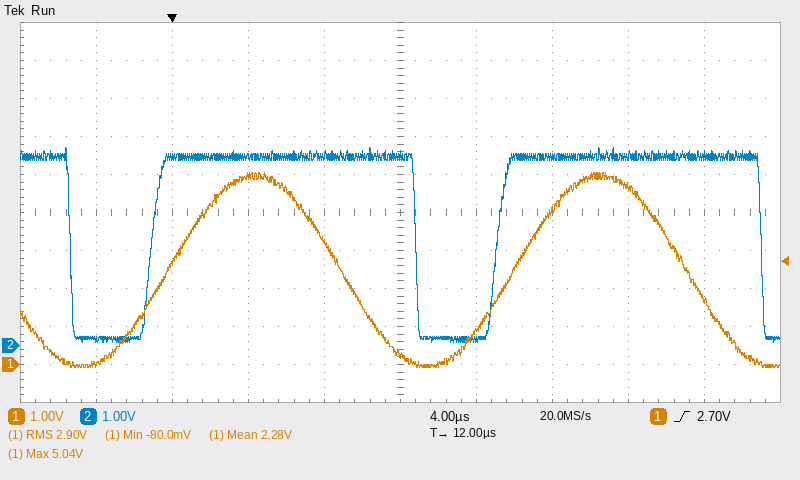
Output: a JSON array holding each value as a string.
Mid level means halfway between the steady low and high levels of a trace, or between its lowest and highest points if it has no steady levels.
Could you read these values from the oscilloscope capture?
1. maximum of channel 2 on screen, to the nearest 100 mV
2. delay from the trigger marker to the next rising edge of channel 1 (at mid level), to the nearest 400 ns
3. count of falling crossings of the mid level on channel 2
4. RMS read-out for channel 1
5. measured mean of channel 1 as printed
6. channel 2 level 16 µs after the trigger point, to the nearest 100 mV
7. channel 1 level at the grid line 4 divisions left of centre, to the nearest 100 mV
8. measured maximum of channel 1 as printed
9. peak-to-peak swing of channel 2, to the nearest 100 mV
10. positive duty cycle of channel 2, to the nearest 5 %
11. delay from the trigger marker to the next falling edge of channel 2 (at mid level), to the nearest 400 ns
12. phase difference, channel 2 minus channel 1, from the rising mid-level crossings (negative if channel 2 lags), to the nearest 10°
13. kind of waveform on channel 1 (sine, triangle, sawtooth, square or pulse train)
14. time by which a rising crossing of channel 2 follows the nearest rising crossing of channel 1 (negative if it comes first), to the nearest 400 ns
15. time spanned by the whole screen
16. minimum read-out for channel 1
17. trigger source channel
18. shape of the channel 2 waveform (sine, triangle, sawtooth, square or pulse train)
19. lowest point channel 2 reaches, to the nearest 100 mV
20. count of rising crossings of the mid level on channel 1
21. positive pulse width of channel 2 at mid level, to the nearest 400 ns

["5.2 V", "18.0 µs", "3", "2.90 V", "2.28 V", "200 mV", "0.0 V", "5.04 V", "5.1 V", "75 %", "12.8 µs", "+20°", "sine", "-800 ns", "40 µs", "-80.0 mV", "channel 1", "pulse train", "100 mV", "2", "14.0 µs"]
